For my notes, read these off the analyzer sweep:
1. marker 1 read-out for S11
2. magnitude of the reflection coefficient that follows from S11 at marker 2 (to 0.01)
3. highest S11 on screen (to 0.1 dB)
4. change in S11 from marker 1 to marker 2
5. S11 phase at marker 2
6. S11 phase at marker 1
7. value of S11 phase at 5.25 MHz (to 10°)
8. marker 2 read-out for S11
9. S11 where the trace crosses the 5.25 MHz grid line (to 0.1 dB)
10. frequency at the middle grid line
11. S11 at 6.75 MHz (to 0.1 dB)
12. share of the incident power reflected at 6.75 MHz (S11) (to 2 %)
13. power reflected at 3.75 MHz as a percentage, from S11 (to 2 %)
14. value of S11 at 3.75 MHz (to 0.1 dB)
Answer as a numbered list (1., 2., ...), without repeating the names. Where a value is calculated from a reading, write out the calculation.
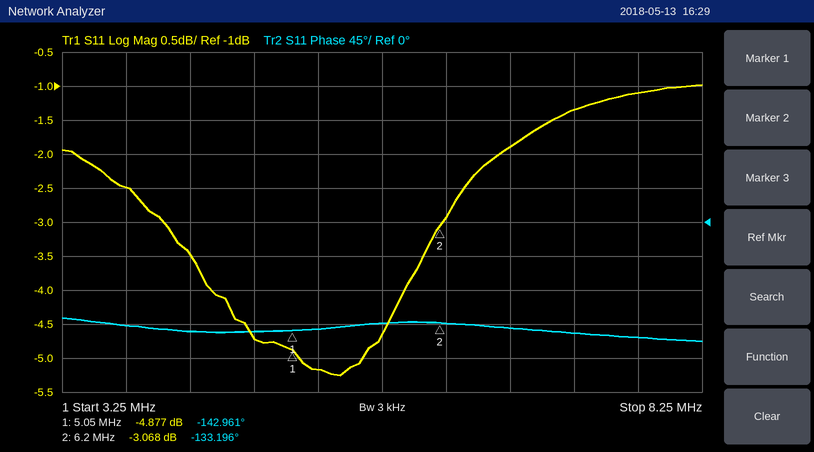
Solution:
1. -4.877 dB
2. 10^(-3.068/20) ≈ 0.70
3. -1.0 dB
4. -3.068 − (-4.877) = 1.809 dB
5. -133.196°
6. -142.961°
7. -140°
8. -3.068 dB
9. -5.2 dB
10. 5.75 MHz
11. -1.9 dB
12. 10^(-1.9/10) ≈ 64.6 %, so 64 % to the nearest 2 %
13. 10^(-2.5/10) ≈ 56 %
14. -2.5 dB
